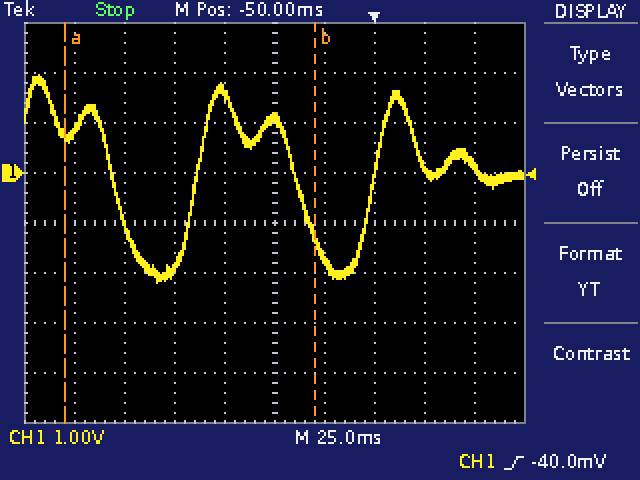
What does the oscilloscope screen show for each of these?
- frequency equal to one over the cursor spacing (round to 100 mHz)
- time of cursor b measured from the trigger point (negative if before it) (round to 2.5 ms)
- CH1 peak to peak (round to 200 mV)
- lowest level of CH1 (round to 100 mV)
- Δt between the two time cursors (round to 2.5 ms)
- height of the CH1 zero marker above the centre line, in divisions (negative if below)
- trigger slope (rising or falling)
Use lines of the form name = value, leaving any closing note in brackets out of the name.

frequency equal to one over the cursor spacing = 8.0 Hz
time of cursor b measured from the trigger point (negative if before it) = -30.0 ms
CH1 peak to peak = 4.2 V
lowest level of CH1 = -2.2 V
Δt between the two time cursors = 125.0 ms
height of the CH1 zero marker above the centre line, in divisions = +1.0 div
trigger slope = rising
